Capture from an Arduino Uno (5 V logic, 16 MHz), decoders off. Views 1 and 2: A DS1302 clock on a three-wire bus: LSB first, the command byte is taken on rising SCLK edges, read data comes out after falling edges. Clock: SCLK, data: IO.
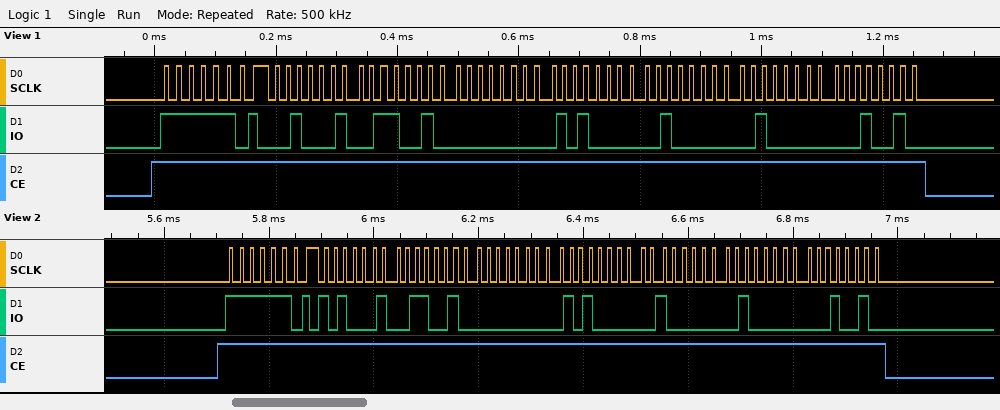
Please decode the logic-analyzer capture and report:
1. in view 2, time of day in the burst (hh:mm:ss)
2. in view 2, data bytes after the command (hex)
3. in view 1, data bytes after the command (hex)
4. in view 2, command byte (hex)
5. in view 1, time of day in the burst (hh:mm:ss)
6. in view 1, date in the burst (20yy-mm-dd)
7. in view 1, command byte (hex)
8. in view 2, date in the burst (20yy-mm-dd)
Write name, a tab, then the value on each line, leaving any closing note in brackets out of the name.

in view 2, time of day in the burst	00:26:45
in view 2, data bytes after the command	45 26 00 05 02 02 24
in view 1, data bytes after the command	44 26 00 05 02 02 24
in view 2, command byte	0xBF
in view 1, time of day in the burst	00:26:44
in view 1, date in the burst	2024-02-05
in view 1, command byte	0xBF
in view 2, date in the burst	2024-02-05
